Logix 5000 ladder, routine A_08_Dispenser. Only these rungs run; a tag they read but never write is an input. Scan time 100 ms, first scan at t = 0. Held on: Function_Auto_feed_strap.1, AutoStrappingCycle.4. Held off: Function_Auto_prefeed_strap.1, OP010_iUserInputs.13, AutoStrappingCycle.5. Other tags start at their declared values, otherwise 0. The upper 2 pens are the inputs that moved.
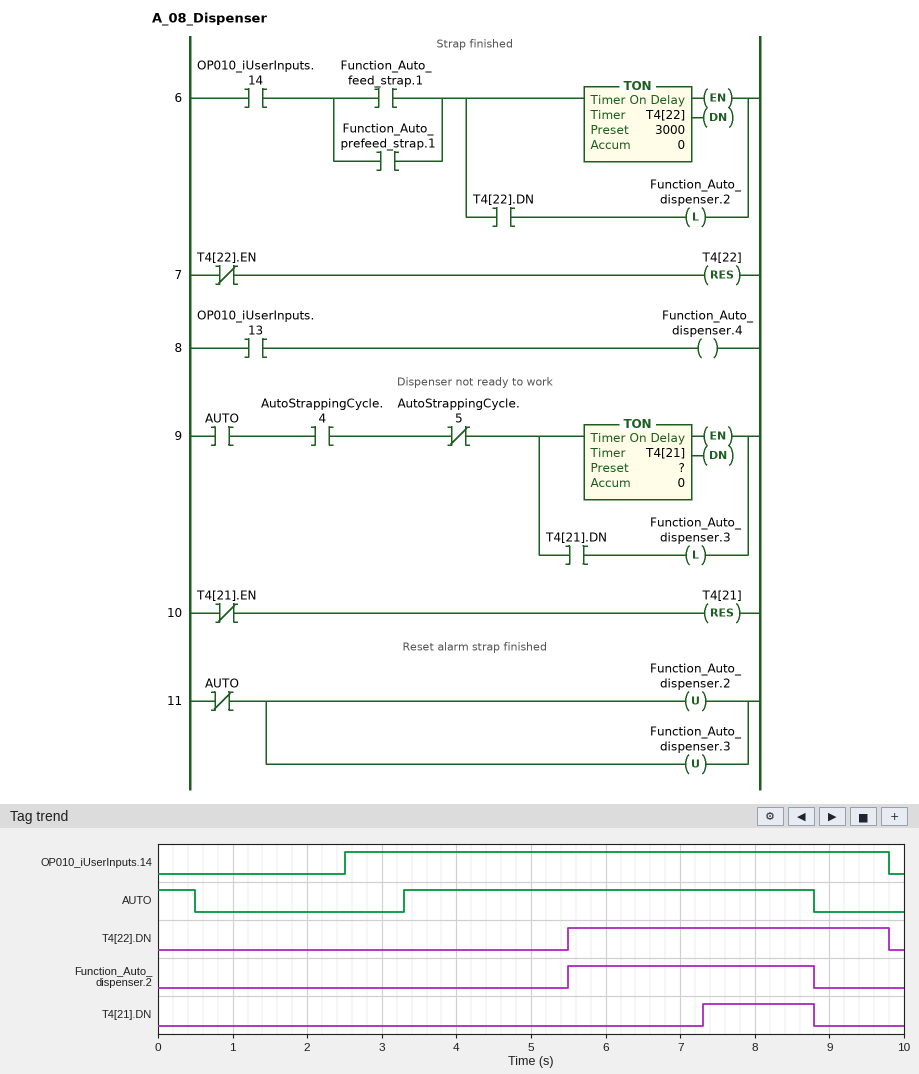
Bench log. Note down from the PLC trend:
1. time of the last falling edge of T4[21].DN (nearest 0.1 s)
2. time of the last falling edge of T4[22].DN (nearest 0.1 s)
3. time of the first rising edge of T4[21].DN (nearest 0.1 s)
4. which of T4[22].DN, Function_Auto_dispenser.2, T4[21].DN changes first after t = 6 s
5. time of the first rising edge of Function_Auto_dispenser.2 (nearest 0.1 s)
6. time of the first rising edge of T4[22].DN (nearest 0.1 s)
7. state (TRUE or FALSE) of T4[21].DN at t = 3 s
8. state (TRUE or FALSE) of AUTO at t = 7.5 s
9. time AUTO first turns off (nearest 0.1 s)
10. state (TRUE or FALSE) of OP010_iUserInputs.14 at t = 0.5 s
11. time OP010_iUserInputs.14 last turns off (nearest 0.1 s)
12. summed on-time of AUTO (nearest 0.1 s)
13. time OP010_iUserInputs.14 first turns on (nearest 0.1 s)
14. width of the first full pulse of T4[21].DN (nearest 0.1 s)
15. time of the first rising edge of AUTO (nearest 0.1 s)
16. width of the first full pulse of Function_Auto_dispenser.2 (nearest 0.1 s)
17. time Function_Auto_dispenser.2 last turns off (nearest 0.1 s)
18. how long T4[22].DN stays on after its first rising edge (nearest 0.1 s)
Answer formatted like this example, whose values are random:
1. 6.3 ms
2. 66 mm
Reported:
1. 8.8 s
2. 9.8 s
3. 7.3 s
4. T4[21].DN
5. 5.5 s
6. 5.5 s
7. FALSE
8. TRUE
9. 0.5 s
10. FALSE
11. 9.8 s
12. 6.0 s
13. 2.5 s
14. 1.5 s
15. 3.3 s
16. 3.3 s
17. 8.8 s
18. 4.3 s
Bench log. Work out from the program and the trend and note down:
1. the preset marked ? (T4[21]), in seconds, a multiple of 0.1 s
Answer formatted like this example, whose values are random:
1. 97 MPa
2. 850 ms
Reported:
1. 4.0 s
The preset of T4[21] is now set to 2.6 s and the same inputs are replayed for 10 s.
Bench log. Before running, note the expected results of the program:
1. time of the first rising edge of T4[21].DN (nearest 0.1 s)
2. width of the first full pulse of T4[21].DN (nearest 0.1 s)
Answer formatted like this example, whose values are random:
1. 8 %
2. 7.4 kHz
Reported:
1. 5.9 s
2. 2.9 s
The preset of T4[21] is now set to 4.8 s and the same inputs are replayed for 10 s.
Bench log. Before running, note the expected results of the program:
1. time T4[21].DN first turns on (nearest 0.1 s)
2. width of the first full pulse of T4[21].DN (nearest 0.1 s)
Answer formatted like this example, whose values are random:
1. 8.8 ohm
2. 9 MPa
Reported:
1. 8.1 s
2. 0.7 s
